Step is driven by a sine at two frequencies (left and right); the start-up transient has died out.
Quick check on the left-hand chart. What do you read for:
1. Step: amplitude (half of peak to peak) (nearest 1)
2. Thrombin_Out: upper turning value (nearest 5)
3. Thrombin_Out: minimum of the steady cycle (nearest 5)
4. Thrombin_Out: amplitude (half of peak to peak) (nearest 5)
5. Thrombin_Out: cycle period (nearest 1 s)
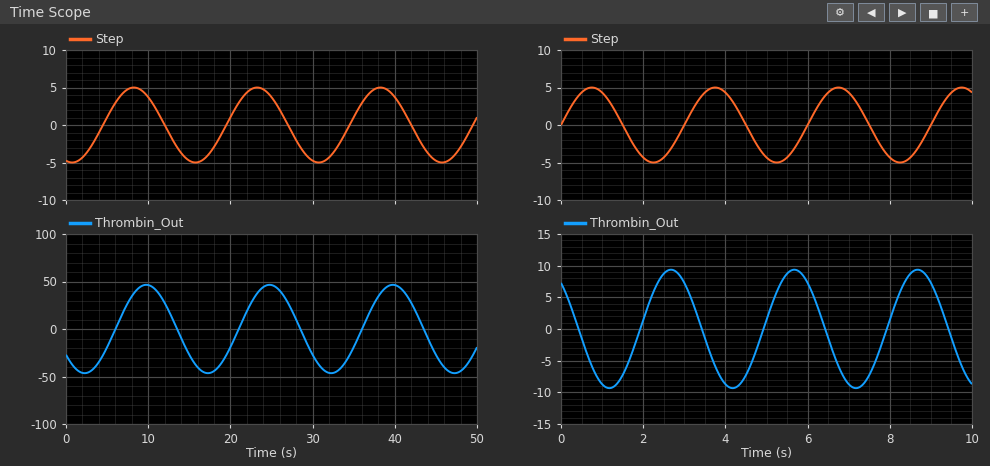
5
45
-45
45
15 s
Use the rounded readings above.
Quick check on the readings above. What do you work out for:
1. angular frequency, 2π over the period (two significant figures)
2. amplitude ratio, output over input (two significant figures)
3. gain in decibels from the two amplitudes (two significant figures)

0.42 rad/s
9.0
19 dB
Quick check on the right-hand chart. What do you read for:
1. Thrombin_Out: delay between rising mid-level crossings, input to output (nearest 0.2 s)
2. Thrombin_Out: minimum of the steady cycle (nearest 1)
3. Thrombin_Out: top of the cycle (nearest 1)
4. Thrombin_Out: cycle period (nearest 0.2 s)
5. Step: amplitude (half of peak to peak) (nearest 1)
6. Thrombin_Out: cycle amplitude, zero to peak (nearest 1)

2.0 s
-9
9
3.0 s
5
9
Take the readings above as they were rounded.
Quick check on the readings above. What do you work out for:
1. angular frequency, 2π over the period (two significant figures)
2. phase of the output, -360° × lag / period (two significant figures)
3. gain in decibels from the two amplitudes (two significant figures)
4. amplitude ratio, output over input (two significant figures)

2.1 rad/s
-240°
5.1 dB
1.8
